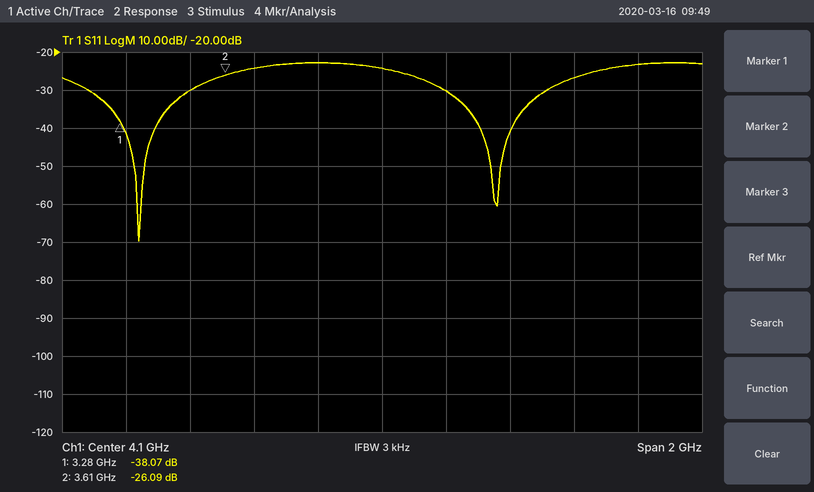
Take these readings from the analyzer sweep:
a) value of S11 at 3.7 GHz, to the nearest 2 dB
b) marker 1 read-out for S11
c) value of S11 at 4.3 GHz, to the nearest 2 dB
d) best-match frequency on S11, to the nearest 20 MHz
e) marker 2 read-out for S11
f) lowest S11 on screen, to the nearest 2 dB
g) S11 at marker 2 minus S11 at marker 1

-24 dB
-38.07 dB
-30 dB
3.34 GHz
-26.09 dB
-70 dB
11.98 dB
